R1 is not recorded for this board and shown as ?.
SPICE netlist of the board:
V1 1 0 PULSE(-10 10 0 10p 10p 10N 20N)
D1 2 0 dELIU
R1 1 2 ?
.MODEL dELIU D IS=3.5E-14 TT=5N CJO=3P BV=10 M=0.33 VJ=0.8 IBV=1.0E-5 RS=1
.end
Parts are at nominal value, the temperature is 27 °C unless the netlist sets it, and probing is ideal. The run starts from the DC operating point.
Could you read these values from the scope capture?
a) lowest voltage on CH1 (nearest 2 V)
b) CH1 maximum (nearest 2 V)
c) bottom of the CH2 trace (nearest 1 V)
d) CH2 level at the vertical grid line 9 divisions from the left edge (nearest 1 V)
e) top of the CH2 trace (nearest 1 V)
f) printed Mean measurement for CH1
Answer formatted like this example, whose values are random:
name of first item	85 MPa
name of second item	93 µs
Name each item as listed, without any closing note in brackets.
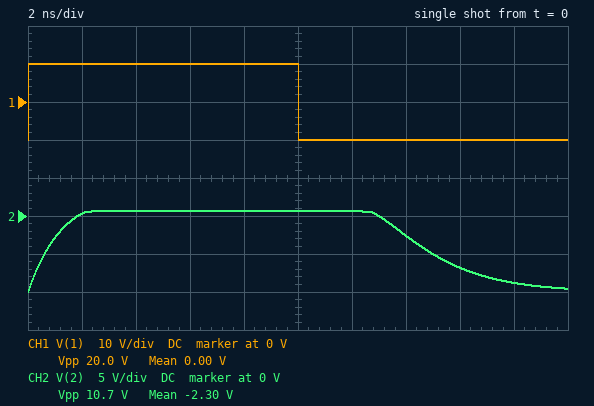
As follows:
lowest voltage on CH1	-10 V
CH1 maximum	10 V
bottom of the CH2 trace	-10 V
CH2 level at the vertical grid line 9 divisions from the left edge	-9 V
top of the CH2 trace	1 V
printed Mean measurement for CH1	0.00 V
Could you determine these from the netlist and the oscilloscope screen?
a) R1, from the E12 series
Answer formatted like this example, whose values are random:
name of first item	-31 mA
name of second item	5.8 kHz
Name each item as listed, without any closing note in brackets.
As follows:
R1, from the E12 series	1.5 kΩ
